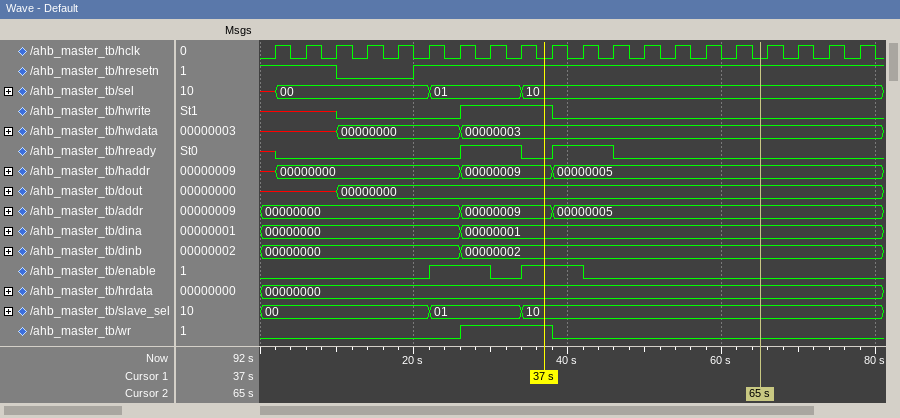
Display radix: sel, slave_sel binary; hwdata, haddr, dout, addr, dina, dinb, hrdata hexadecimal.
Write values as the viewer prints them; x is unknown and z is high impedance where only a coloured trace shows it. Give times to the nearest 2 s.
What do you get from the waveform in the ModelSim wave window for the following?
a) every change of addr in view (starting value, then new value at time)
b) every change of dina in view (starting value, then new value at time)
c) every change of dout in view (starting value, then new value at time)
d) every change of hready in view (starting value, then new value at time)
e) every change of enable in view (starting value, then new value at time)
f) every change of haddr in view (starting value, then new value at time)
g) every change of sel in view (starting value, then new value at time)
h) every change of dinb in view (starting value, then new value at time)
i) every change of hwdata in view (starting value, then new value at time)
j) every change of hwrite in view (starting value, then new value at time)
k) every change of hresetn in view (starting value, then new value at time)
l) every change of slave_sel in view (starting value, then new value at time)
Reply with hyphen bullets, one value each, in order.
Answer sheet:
- 00000000, 00000009 at 26 s, 00000005 at 38 s
- 00000000, 00000001 at 26 s
- x, 00000000 at 10 s
- x, 0 at 2 s, 1 at 26 s, 0 at 34 s, 1 at 38 s, 0 at 46 s
- 0, 1 at 22 s, 0 at 30 s, 1 at 34 s, 0 at 42 s
- x, 00000000 at 2 s, 00000009 at 26 s, 00000005 at 38 s
- x, 00 at 2 s, 01 at 22 s, 10 at 34 s
- 00000000, 00000002 at 26 s
- x, 00000000 at 10 s, 00000003 at 26 s
- x, 0 at 10 s, 1 at 26 s, 0 at 38 s
- 1, 0 at 10 s, 1 at 20 s
- 00, 01 at 22 s, 10 at 34 s
